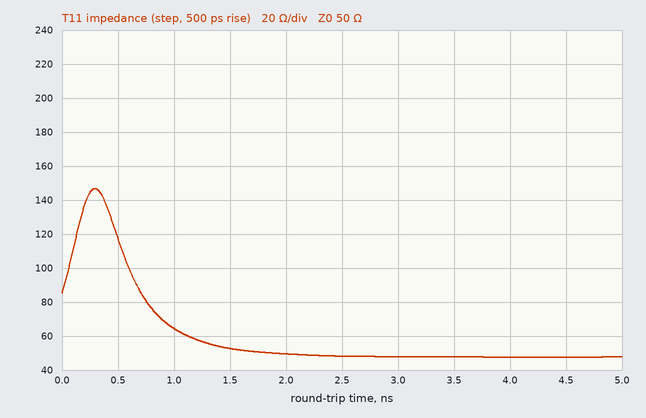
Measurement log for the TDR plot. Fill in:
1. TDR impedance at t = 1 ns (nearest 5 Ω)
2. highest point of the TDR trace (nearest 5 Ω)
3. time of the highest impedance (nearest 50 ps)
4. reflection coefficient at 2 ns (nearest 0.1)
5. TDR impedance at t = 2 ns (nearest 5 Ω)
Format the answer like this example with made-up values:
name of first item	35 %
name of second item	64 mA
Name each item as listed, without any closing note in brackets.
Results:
TDR impedance at t = 1 ns	65 Ω
highest point of the TDR trace	145 Ω
time of the highest impedance	300 ps
reflection coefficient at 2 ns	0.0
TDR impedance at t = 2 ns	50 Ω
